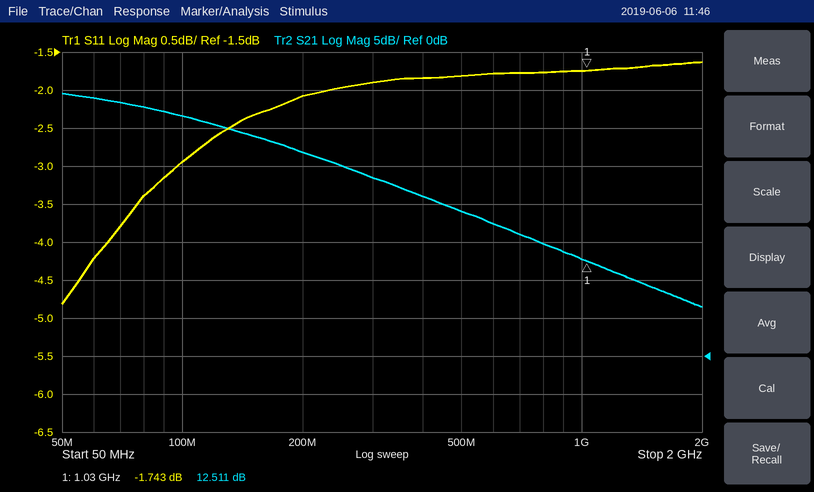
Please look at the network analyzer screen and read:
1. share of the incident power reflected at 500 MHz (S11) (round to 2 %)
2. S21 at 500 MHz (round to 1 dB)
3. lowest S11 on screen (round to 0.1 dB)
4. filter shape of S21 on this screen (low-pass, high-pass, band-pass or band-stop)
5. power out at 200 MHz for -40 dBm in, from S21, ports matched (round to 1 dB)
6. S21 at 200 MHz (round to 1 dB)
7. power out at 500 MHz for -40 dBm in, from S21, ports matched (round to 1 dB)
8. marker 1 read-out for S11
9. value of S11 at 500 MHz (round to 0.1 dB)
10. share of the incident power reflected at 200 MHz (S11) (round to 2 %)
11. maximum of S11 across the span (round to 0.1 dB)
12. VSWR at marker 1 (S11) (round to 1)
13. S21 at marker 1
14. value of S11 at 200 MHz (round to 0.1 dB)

66 %
19 dB
-4.8 dB
low-pass
-13 dBm
27 dB
-21 dBm
-1.743 dB
-1.8 dB
62 %
-1.6 dB
10
12.511 dB
-2.1 dB
